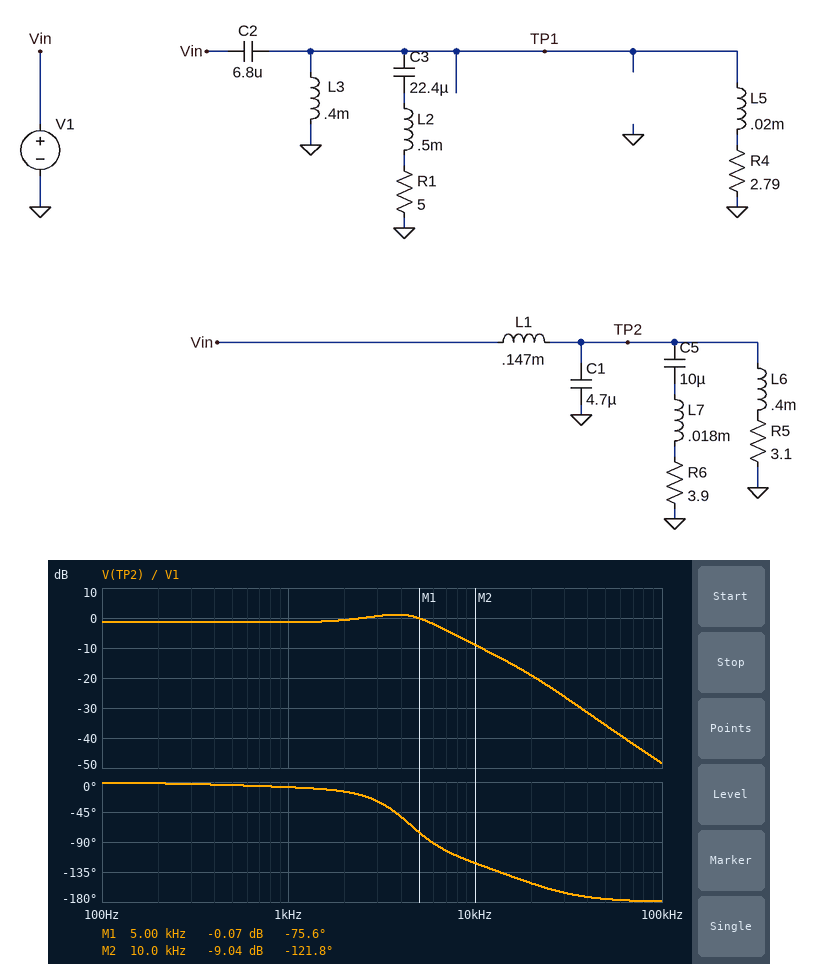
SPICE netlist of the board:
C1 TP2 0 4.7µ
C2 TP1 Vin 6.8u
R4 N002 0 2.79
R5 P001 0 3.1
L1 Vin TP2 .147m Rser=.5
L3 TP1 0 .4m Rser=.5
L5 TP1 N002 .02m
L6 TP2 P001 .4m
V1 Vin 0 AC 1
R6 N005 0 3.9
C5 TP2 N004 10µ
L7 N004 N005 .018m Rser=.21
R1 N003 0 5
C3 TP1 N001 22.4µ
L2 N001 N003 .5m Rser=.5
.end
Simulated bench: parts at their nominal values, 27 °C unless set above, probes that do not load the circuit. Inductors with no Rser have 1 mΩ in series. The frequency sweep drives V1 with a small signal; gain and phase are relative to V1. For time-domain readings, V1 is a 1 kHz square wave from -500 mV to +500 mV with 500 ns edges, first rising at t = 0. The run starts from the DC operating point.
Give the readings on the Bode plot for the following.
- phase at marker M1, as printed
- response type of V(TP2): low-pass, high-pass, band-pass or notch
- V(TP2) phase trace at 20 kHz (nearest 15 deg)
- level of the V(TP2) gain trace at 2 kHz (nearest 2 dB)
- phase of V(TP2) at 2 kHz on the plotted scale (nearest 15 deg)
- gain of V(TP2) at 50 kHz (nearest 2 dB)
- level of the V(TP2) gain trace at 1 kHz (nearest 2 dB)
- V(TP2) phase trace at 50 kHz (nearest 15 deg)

-75.6 deg
low-pass
-150 deg
0 dB
-15 deg
-36 dB
-2 dB
-180 deg
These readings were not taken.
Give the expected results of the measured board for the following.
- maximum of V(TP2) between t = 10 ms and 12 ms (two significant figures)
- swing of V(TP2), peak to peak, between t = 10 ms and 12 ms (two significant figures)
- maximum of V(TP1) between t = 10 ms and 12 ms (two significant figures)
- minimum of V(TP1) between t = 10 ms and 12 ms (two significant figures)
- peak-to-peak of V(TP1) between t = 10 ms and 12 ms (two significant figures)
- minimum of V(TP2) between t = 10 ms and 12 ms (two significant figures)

600 mV
1.2 V
1.0 V
-1.0 V
2.0 V
-600 mV
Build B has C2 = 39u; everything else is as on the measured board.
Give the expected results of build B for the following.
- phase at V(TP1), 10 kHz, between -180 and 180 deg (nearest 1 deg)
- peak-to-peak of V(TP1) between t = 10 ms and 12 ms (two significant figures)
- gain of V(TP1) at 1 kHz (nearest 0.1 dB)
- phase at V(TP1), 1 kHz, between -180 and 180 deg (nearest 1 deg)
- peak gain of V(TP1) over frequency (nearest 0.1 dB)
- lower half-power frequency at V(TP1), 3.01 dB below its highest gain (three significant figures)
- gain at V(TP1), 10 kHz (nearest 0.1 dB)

8 deg
2.1 V
-7.1 dB
97 deg
1.4 dB
1.89 kHz
0.7 dB
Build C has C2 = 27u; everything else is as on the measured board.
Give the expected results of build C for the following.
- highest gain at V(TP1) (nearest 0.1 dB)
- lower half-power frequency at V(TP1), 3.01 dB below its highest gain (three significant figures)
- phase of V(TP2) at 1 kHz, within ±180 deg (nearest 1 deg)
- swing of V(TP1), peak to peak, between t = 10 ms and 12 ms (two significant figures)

1.3 dB
2.37 kHz
-8 deg
2.1 V
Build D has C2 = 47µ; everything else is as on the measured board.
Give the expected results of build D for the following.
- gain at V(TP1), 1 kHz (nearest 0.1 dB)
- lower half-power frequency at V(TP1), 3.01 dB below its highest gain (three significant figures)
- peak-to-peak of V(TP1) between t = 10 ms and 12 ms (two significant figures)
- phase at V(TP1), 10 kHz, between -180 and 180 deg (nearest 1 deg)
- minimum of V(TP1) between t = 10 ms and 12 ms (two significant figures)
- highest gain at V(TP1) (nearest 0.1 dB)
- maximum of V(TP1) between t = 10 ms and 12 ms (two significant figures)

-5.5 dB
1.68 kHz
2.1 V
6 deg
-1.1 V
1.4 dB
1.1 V
